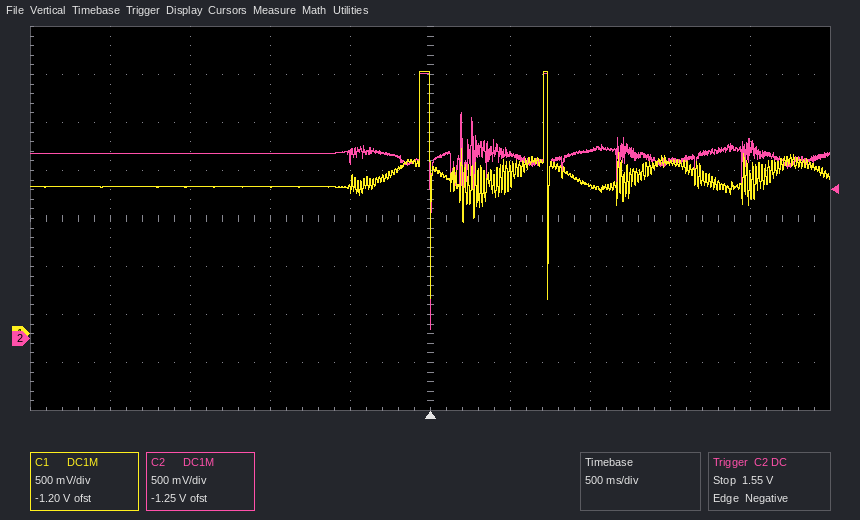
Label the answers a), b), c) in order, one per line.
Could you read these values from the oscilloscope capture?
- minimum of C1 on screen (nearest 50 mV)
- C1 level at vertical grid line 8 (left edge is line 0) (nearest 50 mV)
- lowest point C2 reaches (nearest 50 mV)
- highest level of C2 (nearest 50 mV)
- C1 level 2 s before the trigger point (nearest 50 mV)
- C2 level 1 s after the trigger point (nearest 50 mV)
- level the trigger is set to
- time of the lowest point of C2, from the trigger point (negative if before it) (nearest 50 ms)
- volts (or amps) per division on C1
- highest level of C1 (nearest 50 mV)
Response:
a) 350 mV
b) 1.80 V
c) 100 mV
d) 2.75 V
e) 1.55 V
f) 1.95 V
g) 1.55 V
h) 0 ms
i) 500 mV
j) 2.75 V
